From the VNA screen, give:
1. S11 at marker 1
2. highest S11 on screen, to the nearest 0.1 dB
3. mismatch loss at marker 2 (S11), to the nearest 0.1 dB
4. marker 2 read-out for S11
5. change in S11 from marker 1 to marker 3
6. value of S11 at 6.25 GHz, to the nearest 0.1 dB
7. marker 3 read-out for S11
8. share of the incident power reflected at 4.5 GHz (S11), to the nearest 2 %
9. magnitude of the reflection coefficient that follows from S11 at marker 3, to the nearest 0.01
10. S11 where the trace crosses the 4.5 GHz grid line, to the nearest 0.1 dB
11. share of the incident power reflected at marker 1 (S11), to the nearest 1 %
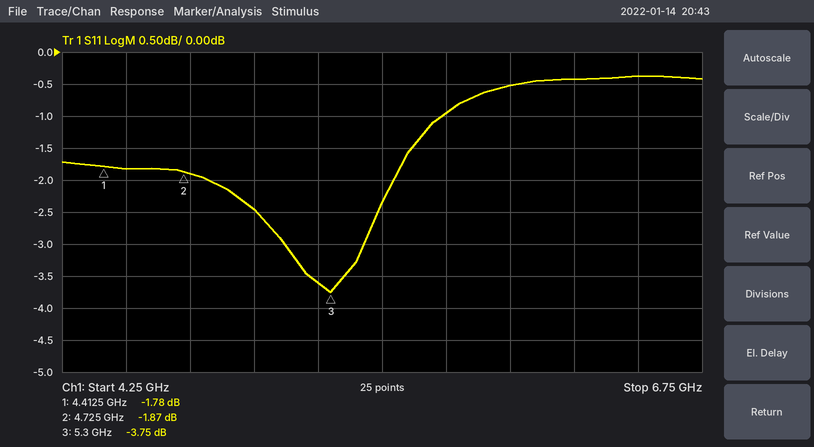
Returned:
-1.78 dB
-0.4 dB
4.6 dB
-1.87 dB
-1.97 dB
-0.4 dB
-3.75 dB
66 %
0.65
-1.8 dB
66 %
